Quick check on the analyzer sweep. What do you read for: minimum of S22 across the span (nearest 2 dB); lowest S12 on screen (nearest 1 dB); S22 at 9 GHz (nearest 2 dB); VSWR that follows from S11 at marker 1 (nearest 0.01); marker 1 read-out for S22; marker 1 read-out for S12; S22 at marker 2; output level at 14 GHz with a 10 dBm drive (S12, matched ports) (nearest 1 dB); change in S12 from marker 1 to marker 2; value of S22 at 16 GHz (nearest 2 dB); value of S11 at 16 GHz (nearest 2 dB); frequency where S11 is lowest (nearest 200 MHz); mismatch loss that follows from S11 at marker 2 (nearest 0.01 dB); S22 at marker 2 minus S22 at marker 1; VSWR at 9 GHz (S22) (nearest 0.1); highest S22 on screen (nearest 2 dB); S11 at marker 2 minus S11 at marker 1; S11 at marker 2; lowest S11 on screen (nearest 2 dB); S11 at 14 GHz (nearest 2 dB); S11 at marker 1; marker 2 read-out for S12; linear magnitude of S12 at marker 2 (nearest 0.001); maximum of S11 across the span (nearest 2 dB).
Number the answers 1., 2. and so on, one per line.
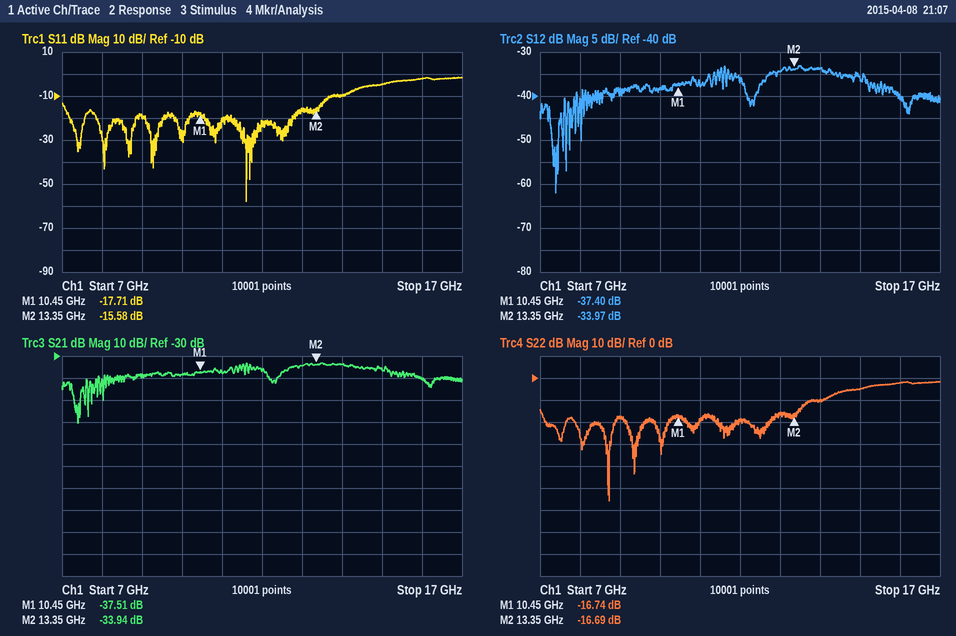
1. -56 dB
2. -62 dB
3. -18 dB
4. 1.30
5. -16.74 dB
6. -37.40 dB
7. -16.69 dB
8. -24 dBm
9. 3.43 dB
10. -2 dB
11. -2 dB
12. 11.6 GHz
13. 0.12 dB
14. 0.05 dB
15. 1.3
16. -2 dB
17. 2.13 dB
18. -15.58 dB
19. -58 dB
20. -10 dB
21. -17.71 dB
22. -33.97 dB
23. 0.020
24. -2 dB
